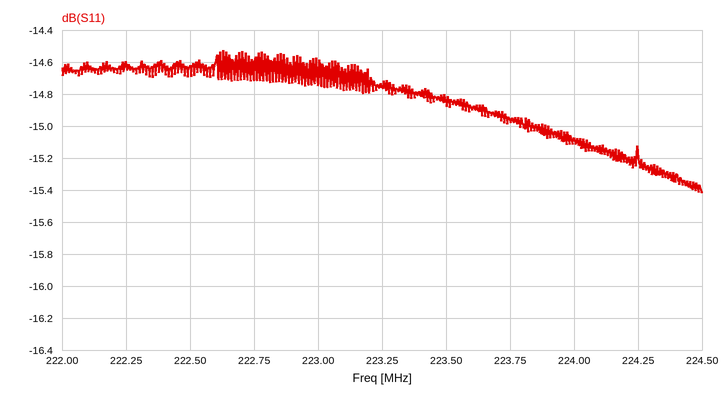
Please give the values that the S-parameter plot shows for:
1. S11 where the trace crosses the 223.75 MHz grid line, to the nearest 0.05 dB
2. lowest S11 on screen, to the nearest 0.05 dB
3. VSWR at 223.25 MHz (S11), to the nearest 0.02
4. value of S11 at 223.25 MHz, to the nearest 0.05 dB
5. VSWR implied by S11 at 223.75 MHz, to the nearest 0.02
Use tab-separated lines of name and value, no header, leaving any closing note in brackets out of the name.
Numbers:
S11 where the trace crosses the 223.75 MHz grid line, to the nearest 0.05 dB	-14.95 dB
lowest S11 on screen, to the nearest 0.05 dB	-15.40 dB
VSWR at 223.25 MHz (S11), to the nearest 0.02	1.44
value of S11 at 223.25 MHz, to the nearest 0.05 dB	-14.75 dB
VSWR implied by S11 at 223.75 MHz, to the nearest 0.02	1.44
